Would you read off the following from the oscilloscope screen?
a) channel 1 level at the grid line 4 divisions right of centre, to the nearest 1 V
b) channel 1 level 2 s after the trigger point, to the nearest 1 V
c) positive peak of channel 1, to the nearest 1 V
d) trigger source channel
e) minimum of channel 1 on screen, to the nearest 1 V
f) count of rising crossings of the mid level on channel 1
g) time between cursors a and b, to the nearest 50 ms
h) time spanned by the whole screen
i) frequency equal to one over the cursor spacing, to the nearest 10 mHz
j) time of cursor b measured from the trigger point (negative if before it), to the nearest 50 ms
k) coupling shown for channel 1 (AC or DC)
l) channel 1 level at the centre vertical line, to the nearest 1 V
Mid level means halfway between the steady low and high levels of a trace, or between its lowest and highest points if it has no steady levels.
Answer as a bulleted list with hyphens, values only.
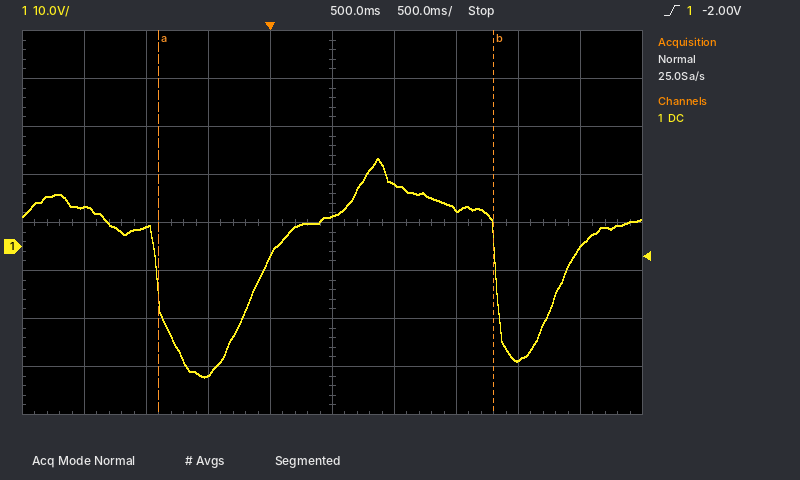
- 0 V
- -24 V
- 18 V
- channel 1
- -27 V
- 2
- 2.70 s
- 5 s
- 370 mHz
- +1.80 s
- DC
- 6 V
